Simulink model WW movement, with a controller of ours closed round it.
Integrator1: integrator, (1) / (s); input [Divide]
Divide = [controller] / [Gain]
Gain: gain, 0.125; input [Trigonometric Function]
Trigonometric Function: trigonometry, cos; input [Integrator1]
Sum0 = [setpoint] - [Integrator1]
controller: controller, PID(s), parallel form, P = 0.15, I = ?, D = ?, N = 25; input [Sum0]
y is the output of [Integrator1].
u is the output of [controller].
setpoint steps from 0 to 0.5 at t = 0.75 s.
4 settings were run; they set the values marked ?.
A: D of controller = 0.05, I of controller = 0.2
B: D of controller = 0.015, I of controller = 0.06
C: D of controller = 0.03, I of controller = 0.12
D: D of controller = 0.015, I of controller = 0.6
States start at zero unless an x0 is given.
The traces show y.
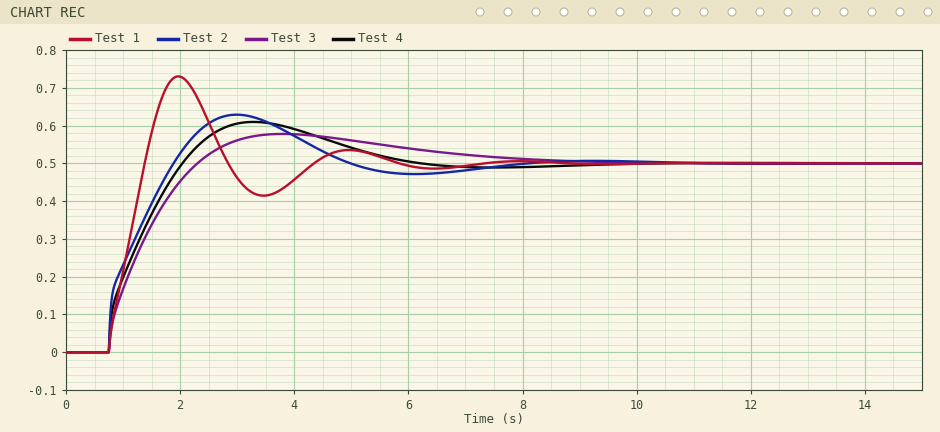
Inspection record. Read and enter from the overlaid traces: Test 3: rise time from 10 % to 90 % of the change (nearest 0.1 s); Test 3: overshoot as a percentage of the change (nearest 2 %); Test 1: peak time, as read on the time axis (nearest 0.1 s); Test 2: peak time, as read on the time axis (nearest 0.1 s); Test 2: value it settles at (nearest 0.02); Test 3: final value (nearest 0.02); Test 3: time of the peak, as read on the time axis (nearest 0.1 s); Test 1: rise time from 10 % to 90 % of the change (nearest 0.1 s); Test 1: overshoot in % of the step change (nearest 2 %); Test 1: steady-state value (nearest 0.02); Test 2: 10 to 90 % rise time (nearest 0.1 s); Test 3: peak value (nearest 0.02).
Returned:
1.2 s
16 %
2.0 s
3.0 s
0.50
0.50
3.8 s
0.5 s
46 %
0.50
0.9 s
0.58
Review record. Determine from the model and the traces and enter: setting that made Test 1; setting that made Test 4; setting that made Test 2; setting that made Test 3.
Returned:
D
C
A
B
